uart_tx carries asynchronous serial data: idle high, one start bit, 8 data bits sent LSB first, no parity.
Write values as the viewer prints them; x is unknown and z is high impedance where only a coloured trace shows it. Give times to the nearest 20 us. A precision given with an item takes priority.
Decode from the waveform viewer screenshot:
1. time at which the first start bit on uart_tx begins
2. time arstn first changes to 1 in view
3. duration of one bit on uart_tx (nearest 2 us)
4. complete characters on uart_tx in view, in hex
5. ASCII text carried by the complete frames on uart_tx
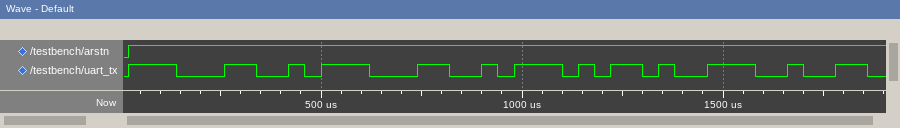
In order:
140 us
20 us
40 us
4C, 4C, 2D
"LL-"
